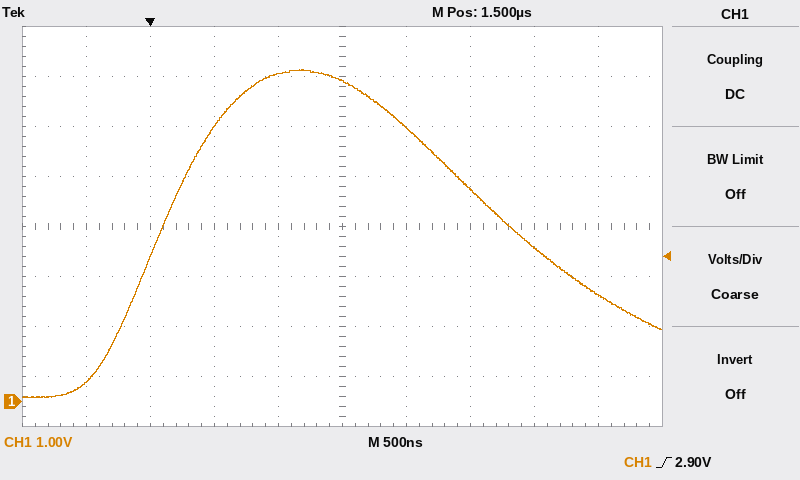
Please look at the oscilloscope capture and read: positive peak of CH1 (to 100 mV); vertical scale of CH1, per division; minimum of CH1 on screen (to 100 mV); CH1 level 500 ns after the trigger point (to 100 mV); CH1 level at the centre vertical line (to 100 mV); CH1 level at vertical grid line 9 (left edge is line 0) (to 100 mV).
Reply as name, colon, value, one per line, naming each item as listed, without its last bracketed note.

positive peak of CH1: 6.6 V
vertical scale of CH1, per division: 1 V
minimum of CH1 on screen: 100 mV
CH1 level 500 ns after the trigger point: 5.5 V
CH1 level at the centre vertical line: 6.4 V
CH1 level at vertical grid line 9 (left edge is line 0): 2.1 V
